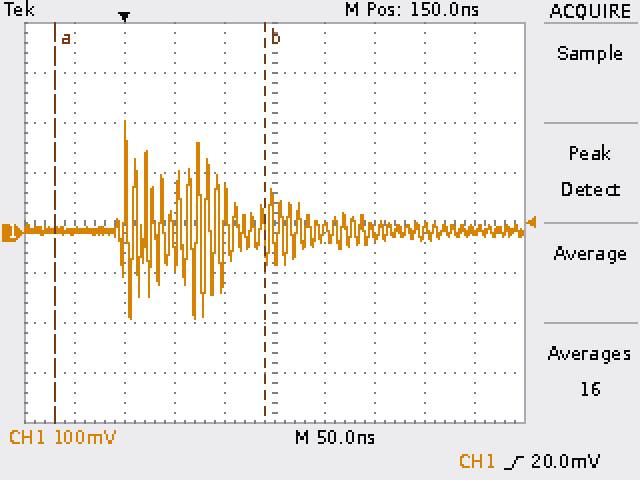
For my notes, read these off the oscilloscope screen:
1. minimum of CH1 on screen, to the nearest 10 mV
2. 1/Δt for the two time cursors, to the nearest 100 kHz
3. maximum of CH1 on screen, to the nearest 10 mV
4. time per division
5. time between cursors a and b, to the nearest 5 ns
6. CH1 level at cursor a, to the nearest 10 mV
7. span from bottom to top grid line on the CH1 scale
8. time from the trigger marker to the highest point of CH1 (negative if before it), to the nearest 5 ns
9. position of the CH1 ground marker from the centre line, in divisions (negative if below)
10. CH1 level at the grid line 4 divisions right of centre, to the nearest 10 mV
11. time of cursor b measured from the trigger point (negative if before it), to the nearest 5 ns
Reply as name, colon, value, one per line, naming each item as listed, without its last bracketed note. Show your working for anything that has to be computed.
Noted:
minimum of CH1 on screen, to the nearest 10 mV: -170 mV
1/Δt for the two time cursors, to the nearest 100 kHz: 1 / 210 ns ≈ 4.8 MHz
maximum of CH1 on screen, to the nearest 10 mV: 220 mV
time per division: 50 ns
time between cursors a and b, to the nearest 5 ns: 210 ns
CH1 level at cursor a, to the nearest 10 mV: 10 mV
span from bottom to top grid line on the CH1 scale: 800 mV
time from the trigger marker to the highest point of CH1 (negative if before it), to the nearest 5 ns: 0 ns
position of the CH1 ground marker from the centre line, in divisions: -0.2 div
CH1 level at the grid line 4 divisions right of centre, to the nearest 10 mV: 10 mV
time of cursor b measured from the trigger point (negative if before it), to the nearest 5 ns: +140 ns
